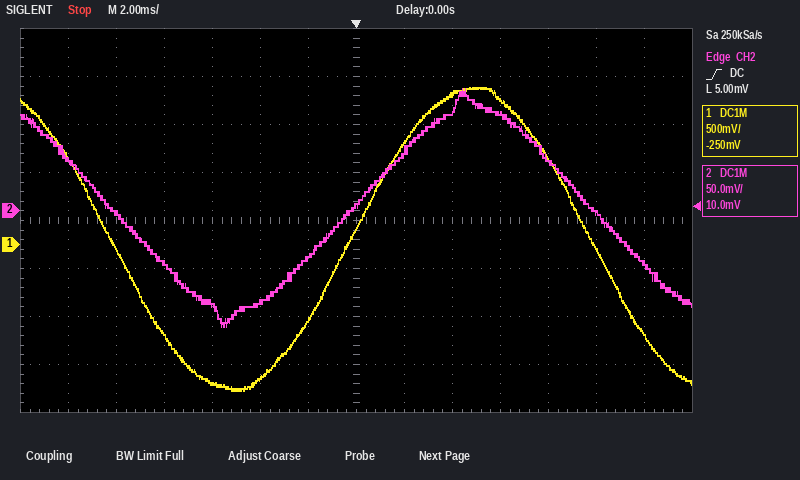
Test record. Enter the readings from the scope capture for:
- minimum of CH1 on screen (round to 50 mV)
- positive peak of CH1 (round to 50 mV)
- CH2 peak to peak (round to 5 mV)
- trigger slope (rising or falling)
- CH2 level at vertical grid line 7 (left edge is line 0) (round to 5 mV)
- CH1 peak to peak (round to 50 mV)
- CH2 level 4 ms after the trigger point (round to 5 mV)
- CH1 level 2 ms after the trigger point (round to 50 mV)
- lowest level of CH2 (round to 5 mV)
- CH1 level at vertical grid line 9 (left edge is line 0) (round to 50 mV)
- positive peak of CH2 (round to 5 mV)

-1.50 V
1.65 V
250 mV
rising
5 mV
3.15 V
105 mV
1.05 V
-120 mV
1.55 V
130 mV
